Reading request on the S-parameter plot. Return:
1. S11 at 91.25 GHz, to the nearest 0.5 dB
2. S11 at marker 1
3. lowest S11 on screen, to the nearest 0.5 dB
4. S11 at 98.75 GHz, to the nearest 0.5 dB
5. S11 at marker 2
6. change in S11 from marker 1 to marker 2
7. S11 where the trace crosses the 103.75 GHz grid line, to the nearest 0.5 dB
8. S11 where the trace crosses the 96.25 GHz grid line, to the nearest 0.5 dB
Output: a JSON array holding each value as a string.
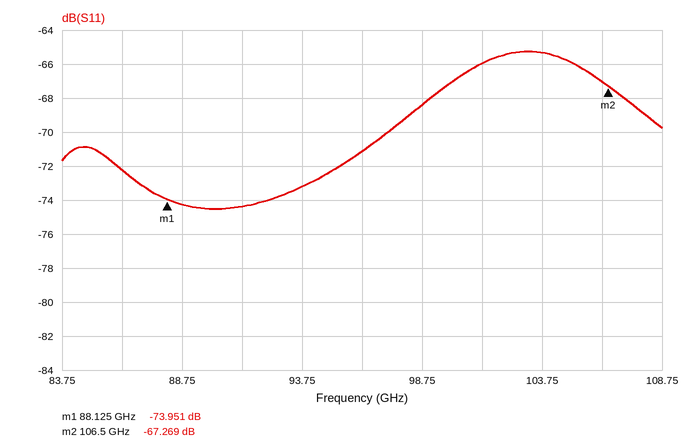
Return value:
["-74.5 dB", "-73.951 dB", "-74.5 dB", "-68.5 dB", "-67.269 dB", "6.682 dB", "-65.5 dB", "-71.0 dB"]
